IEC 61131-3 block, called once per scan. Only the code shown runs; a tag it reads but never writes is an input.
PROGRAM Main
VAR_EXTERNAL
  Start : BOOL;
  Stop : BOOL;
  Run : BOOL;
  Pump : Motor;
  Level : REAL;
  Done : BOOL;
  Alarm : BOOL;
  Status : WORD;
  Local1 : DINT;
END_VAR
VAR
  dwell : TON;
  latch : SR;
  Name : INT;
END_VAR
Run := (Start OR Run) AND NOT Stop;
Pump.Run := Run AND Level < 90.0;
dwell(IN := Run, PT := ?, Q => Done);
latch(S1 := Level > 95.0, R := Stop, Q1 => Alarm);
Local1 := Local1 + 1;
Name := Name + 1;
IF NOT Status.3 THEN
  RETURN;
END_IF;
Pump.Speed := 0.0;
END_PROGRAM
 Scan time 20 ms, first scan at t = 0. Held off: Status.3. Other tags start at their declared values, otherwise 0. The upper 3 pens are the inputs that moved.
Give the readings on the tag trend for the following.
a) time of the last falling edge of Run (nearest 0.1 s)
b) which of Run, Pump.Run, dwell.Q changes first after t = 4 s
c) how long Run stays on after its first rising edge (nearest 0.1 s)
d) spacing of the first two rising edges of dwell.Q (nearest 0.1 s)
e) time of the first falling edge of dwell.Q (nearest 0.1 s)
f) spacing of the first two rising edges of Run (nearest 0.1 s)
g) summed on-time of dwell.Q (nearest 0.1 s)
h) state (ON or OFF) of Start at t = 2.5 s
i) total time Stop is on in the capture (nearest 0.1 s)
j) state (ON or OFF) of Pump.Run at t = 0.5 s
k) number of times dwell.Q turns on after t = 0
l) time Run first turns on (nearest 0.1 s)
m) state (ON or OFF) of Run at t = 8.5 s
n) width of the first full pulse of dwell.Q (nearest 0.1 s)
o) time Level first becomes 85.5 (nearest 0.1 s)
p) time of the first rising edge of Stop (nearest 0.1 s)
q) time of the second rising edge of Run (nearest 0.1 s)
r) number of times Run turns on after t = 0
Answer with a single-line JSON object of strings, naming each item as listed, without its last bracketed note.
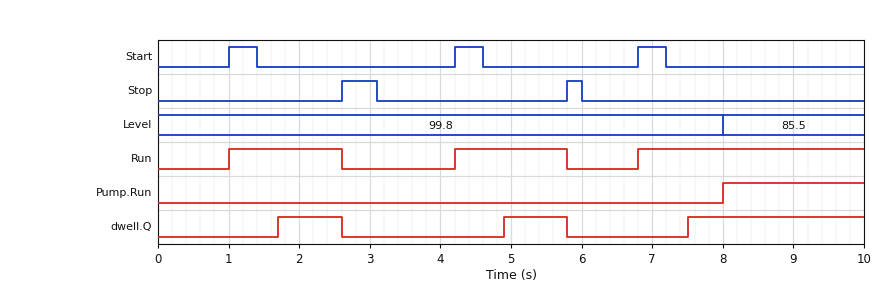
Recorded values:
{"time of the last falling edge of Run": "5.8 s", "which of Run, Pump.Run, dwell.Q changes first after t = 4 s": "Run", "how long Run stays on after its first rising edge": "1.6 s", "spacing of the first two rising edges of dwell.Q": "3.2 s", "time of the first falling edge of dwell.Q": "2.6 s", "spacing of the first two rising edges of Run": "3.2 s", "summed on-time of dwell.Q": "4.3 s", "state (ON or OFF) of Start at t = 2.5 s": "OFF", "total time Stop is on in the capture": "0.7 s", "state (ON or OFF) of Pump.Run at t = 0.5 s": "OFF", "number of times dwell.Q turns on after t = 0": "3", "time Run first turns on": "1.0 s", "state (ON or OFF) of Run at t = 8.5 s": "ON", "width of the first full pulse of dwell.Q": "0.9 s", "time Level first becomes 85.5": "8.0 s", "time of the first rising edge of Stop": "2.6 s", "time of the second rising edge of Run": "4.2 s", "number of times Run turns on after t = 0": "3"}
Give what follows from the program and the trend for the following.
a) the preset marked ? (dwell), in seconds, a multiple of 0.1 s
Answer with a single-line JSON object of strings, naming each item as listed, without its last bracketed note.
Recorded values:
{"the preset marked ? (dwell), in seconds, a multiple of 0.1 s": "0.7 s"}
